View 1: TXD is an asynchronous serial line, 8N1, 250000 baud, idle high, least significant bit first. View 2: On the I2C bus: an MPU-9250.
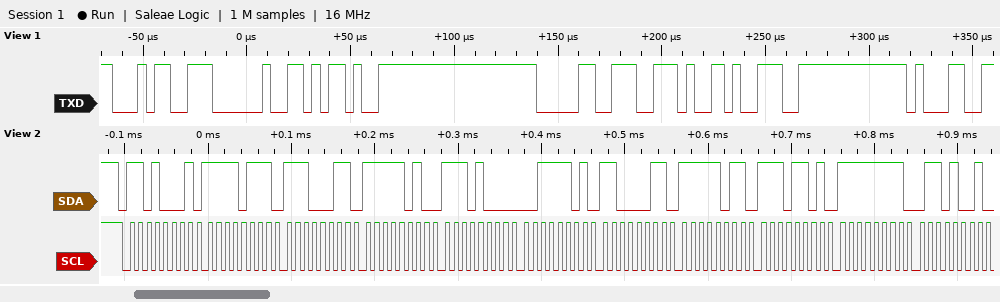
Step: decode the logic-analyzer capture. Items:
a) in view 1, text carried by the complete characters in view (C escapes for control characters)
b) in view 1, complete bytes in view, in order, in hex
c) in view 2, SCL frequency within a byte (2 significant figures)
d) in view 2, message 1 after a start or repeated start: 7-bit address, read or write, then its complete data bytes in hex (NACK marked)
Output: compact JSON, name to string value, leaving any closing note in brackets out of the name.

{"in view 1, text carried by the complete characters in view": "\"4 -0.91\"", "in view 1, complete bytes in view, in order, in hex": "0x34 0x20 0x2D 0x30 0x2E 0x39 0x31", "in view 2, SCL frequency within a byte": "100 kHz", "in view 2, message 1 after a start or repeated start: 7-bit address, read or write, then its complete data bytes in hex": "0x68 read: F7 E3 FA E8 3D C3 FB ED FF 69"}
